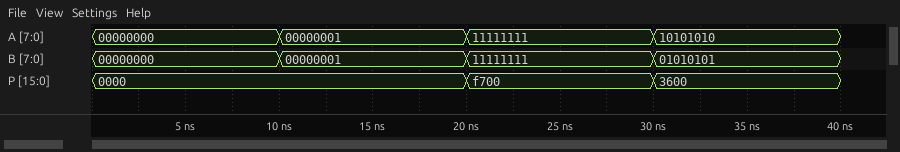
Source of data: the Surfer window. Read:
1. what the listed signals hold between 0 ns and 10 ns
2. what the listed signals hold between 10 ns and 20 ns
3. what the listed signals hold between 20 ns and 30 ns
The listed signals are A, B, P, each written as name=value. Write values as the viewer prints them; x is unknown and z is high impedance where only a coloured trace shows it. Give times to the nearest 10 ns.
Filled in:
A=00000000, B=00000000, P=0000
A=00000001, B=00000001, P=0000
A=11111111, B=11111111, P=f700
